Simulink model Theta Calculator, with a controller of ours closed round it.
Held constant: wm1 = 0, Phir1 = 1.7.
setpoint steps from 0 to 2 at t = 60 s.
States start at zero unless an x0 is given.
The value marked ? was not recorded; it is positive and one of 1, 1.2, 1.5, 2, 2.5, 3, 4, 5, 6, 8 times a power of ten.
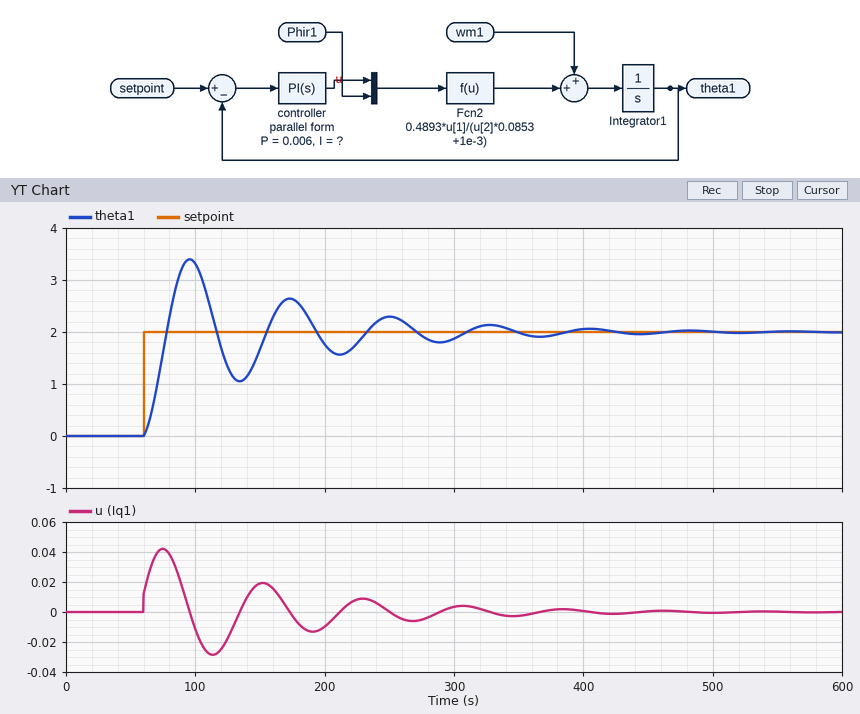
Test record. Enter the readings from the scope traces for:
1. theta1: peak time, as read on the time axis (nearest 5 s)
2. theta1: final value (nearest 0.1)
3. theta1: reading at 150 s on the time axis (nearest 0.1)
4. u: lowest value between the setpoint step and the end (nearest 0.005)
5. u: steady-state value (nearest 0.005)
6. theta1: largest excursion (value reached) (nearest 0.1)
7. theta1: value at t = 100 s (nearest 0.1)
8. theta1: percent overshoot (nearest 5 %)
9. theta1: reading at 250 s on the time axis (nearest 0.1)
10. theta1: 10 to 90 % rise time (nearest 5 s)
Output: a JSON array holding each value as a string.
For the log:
["95 s", "2.0", "1.7", "-0.030", "0.000", "3.4", "3.3", "70 %", "2.3", "15 s"]
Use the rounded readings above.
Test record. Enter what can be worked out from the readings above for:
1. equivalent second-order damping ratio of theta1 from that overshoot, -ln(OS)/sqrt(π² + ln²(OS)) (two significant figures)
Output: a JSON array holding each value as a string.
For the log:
["0.11"]
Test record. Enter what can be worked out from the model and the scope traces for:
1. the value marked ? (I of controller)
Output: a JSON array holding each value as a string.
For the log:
["0.002"]
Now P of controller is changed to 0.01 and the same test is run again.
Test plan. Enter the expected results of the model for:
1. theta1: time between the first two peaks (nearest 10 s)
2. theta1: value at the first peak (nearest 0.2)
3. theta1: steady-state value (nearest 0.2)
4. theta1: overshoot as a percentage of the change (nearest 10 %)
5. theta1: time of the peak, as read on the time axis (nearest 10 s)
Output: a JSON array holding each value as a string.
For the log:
["80 s", "3.2", "2.0", "60 %", "90 s"]
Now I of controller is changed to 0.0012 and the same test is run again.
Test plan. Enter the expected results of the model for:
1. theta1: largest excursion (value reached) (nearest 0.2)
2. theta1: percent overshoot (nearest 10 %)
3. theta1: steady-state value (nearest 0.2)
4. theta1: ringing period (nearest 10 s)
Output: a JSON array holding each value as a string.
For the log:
["3.2", "60 %", "2.0", "100 s"]
